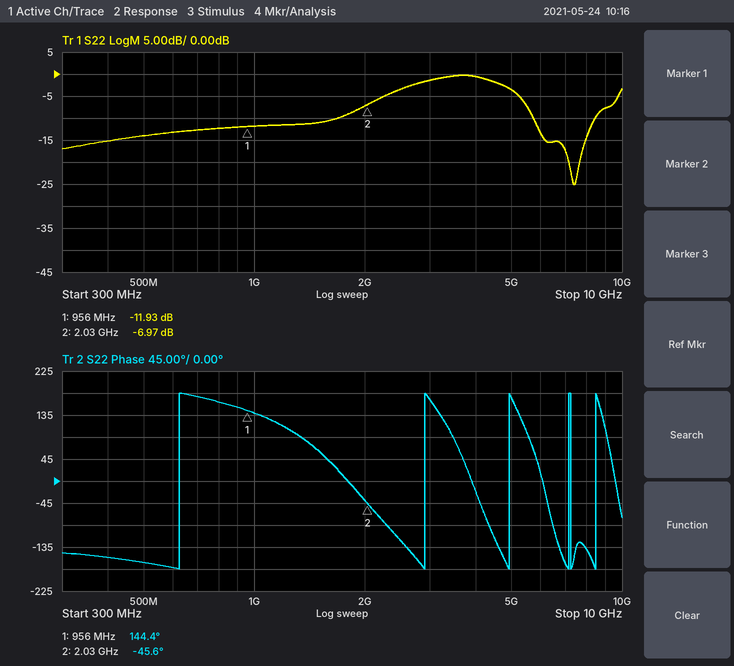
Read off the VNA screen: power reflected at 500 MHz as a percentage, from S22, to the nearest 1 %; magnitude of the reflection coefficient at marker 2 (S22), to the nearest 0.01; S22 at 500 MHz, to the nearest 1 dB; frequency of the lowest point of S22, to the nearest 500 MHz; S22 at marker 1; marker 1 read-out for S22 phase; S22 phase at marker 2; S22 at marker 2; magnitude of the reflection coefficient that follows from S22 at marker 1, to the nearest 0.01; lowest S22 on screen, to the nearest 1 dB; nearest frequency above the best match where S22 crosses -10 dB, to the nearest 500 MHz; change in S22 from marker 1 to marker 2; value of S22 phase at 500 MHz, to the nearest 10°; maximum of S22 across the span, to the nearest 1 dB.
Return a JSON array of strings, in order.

["4 %", "0.45", "-14 dB", "7.5 GHz", "-11.93 dB", "144.4°", "-45.6°", "-6.97 dB", "0.25", "-25 dB", "8.5 GHz", "4.96 dB", "-170°", "0 dB"]
